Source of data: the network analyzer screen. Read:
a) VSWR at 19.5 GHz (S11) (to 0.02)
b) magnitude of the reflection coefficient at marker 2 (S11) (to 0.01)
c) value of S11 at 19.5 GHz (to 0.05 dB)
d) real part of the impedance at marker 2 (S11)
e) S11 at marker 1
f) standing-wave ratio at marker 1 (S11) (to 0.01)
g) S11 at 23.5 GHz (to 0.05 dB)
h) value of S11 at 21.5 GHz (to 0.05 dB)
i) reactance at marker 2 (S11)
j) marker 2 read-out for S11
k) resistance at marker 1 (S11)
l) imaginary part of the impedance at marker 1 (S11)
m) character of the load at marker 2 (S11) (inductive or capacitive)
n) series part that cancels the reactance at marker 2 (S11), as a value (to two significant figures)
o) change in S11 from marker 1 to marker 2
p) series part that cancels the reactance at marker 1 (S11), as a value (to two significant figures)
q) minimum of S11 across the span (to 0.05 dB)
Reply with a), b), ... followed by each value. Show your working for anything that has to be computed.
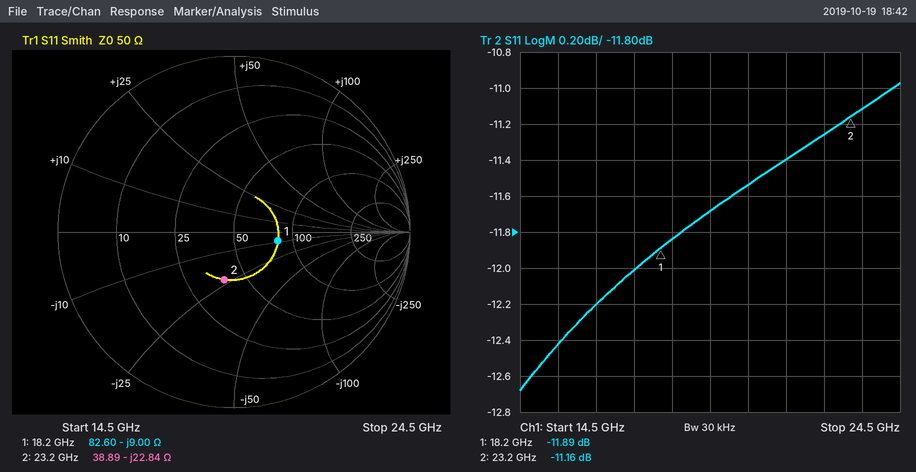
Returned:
a) |Γ| = 10^(-11.7/20) = 0.2600; VSWR = (1 + 0.2600)/(1 − 0.2600) ≈ 1.70
b) 0.28
c) -11.70 dB
d) 38.89 Ω
e) -11.89 dB
f) 1.68
g) -11.10 dB
h) -11.40 dB
i) -22.84 Ω
j) -11.16 dB
k) 82.60 Ω
l) -9.00 Ω
m) capacitive
n) L = 22.84 Ω/(2π × 23.2 GHz) ≈ 157 pH, so 160 pH to two significant figures
o) -11.16 − (-11.89) = 0.73 dB
p) L = 9 Ω/(2π × 18.2 GHz) ≈ 79 pH
q) -12.70 dB
